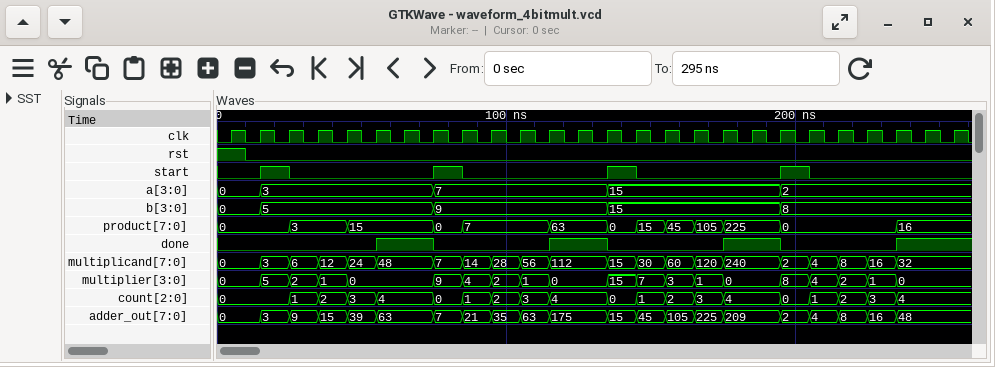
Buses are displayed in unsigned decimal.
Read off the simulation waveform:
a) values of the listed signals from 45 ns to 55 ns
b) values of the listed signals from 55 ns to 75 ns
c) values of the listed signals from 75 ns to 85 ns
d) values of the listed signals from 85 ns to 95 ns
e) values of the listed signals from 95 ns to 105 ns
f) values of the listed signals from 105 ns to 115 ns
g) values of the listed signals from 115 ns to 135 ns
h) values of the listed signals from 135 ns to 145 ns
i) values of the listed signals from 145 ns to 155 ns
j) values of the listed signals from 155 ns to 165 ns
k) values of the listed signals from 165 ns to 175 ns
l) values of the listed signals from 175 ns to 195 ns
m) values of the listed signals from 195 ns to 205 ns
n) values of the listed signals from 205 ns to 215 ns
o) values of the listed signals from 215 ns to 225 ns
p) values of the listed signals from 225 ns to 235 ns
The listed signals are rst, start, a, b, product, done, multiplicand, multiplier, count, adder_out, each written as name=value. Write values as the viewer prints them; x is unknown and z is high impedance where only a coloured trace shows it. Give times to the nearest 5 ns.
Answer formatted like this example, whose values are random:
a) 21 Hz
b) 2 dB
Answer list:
a) rst=0, start=0, a=3, b=5, product=15, done=0, multiplicand=24, multiplier=0, count=3, adder_out=39
b) rst=0, start=0, a=3, b=5, product=15, done=1, multiplicand=48, multiplier=0, count=4, adder_out=63
c) rst=0, start=1, a=7, b=9, product=0, done=0, multiplicand=7, multiplier=9, count=0, adder_out=7
d) rst=0, start=0, a=7, b=9, product=7, done=0, multiplicand=14, multiplier=4, count=1, adder_out=21
e) rst=0, start=0, a=7, b=9, product=7, done=0, multiplicand=28, multiplier=2, count=2, adder_out=35
f) rst=0, start=0, a=7, b=9, product=7, done=0, multiplicand=56, multiplier=1, count=3, adder_out=63
g) rst=0, start=0, a=7, b=9, product=63, done=1, multiplicand=112, multiplier=0, count=4, adder_out=175
h) rst=0, start=1, a=15, b=15, product=0, done=0, multiplicand=15, multiplier=15, count=0, adder_out=15
i) rst=0, start=0, a=15, b=15, product=15, done=0, multiplicand=30, multiplier=7, count=1, adder_out=45
j) rst=0, start=0, a=15, b=15, product=45, done=0, multiplicand=60, multiplier=3, count=2, adder_out=105
k) rst=0, start=0, a=15, b=15, product=105, done=0, multiplicand=120, multiplier=1, count=3, adder_out=225
l) rst=0, start=0, a=15, b=15, product=225, done=1, multiplicand=240, multiplier=0, count=4, adder_out=209
m) rst=0, start=1, a=2, b=8, product=0, done=0, multiplicand=2, multiplier=8, count=0, adder_out=2
n) rst=0, start=0, a=2, b=8, product=0, done=0, multiplicand=4, multiplier=4, count=1, adder_out=4
o) rst=0, start=0, a=2, b=8, product=0, done=0, multiplicand=8, multiplier=2, count=2, adder_out=8
p) rst=0, start=0, a=2, b=8, product=0, done=0, multiplicand=16, multiplier=1, count=3, adder_out=16
